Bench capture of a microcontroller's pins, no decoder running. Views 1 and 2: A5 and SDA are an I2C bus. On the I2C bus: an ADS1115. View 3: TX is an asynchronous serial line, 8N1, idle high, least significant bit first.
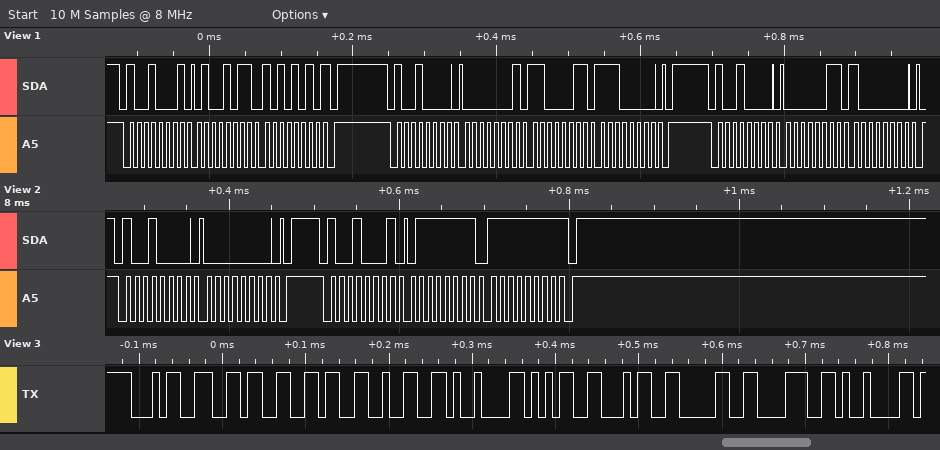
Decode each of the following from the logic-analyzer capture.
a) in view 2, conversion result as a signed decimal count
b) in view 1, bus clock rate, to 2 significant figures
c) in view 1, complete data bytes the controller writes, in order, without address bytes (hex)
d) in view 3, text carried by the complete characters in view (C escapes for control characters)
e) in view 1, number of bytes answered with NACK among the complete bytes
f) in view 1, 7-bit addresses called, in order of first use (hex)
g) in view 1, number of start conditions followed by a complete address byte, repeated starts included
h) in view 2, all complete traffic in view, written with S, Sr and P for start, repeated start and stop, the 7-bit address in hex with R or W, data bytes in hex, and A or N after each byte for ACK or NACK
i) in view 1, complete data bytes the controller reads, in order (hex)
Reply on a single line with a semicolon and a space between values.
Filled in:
32767; 100 kHz; 01 C3 E0 03 80; "4662\t5408\t"; 1; 0x48; 3; S 48W A 00 A P S 48R A 7F A FF N P; 4B AA
